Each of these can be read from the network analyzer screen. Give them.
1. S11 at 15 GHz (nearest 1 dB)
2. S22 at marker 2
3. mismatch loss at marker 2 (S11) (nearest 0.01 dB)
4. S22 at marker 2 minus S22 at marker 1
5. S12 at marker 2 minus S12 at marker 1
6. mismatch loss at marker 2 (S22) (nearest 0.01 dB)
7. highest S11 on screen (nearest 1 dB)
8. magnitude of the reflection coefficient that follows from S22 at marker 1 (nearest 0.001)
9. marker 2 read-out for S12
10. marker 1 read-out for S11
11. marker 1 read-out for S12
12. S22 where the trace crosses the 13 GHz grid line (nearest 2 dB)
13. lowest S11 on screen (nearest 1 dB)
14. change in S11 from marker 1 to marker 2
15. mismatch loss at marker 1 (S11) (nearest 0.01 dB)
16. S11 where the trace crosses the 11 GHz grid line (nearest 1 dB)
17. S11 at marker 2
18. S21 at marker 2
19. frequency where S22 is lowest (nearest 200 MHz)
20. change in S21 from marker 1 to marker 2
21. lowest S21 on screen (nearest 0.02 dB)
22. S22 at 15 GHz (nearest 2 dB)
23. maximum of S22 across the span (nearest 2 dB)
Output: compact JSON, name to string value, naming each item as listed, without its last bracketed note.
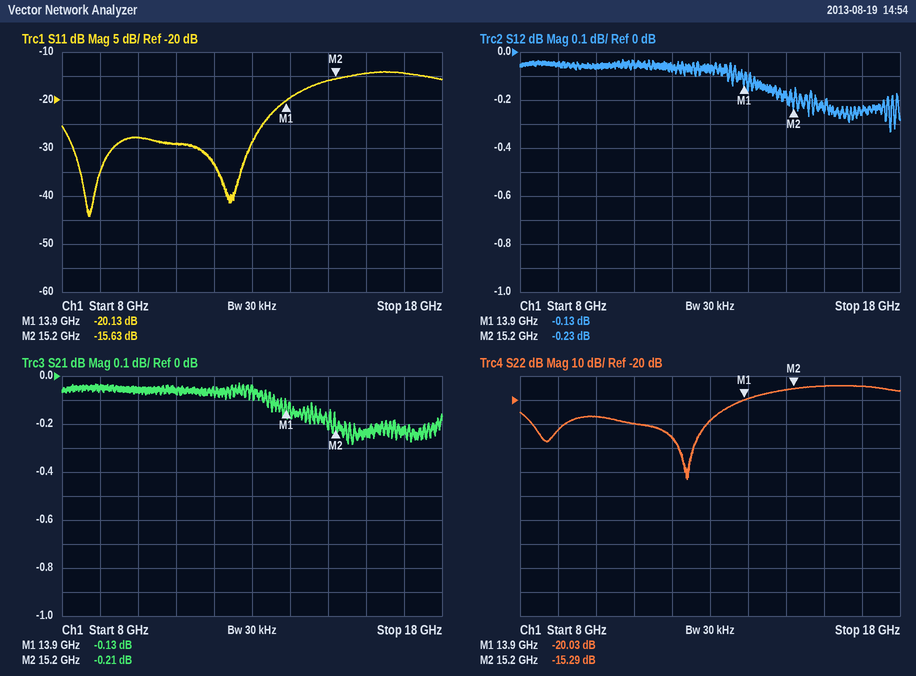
{"S11 at 15 GHz": "-16 dB", "S22 at marker 2": "-15.29 dB", "mismatch loss at marker 2 (S11)": "0.12 dB", "S22 at marker 2 minus S22 at marker 1": "4.74 dB", "S12 at marker 2 minus S12 at marker 1": "-0.10 dB", "mismatch loss at marker 2 (S22)": "0.13 dB", "highest S11 on screen": "-14 dB", "magnitude of the reflection coefficient that follows from S22 at marker 1": "0.100", "marker 2 read-out for S12": "-0.23 dB", "marker 1 read-out for S11": "-20.13 dB", "marker 1 read-out for S12": "-0.13 dB", "S22 where the trace crosses the 13 GHz grid line": "-28 dB", "lowest S11 on screen": "-44 dB", "change in S11 from marker 1 to marker 2": "4.50 dB", "mismatch loss at marker 1 (S11)": "0.04 dB", "S11 where the trace crosses the 11 GHz grid line": "-29 dB", "S11 at marker 2": "-15.63 dB", "S21 at marker 2": "-0.21 dB", "frequency where S22 is lowest": "12.4 GHz", "change in S21 from marker 1 to marker 2": "-0.08 dB", "lowest S21 on screen": "-0.28 dB", "S22 at 15 GHz": "-16 dB", "maximum of S22 across the span": "-14 dB"}
